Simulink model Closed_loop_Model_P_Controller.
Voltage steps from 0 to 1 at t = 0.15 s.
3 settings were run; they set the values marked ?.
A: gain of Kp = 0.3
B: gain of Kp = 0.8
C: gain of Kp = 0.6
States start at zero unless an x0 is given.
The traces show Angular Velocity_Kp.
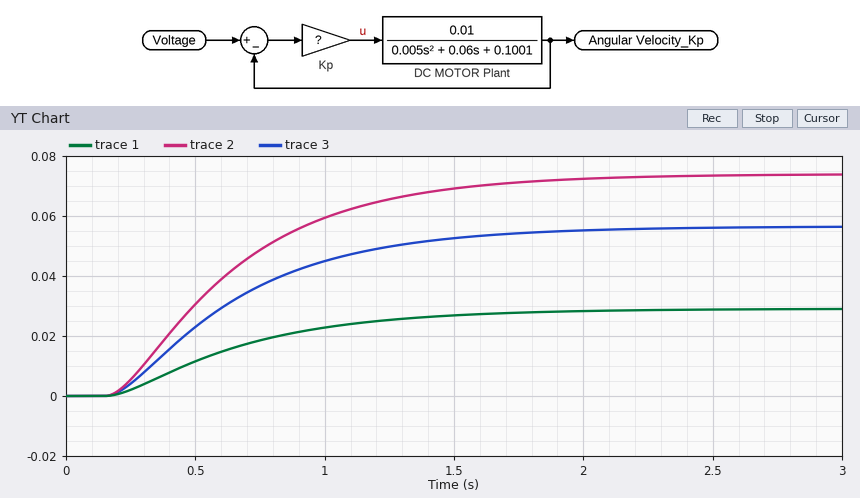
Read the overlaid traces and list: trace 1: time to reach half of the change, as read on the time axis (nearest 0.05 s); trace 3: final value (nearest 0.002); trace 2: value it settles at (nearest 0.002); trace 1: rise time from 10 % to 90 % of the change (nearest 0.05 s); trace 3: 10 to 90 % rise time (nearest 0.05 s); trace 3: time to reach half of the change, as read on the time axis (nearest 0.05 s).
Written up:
0.60 s
0.056
0.074
1.10 s
1.05 s
0.60 s
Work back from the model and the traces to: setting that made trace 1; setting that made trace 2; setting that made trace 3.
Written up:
A
B
C
